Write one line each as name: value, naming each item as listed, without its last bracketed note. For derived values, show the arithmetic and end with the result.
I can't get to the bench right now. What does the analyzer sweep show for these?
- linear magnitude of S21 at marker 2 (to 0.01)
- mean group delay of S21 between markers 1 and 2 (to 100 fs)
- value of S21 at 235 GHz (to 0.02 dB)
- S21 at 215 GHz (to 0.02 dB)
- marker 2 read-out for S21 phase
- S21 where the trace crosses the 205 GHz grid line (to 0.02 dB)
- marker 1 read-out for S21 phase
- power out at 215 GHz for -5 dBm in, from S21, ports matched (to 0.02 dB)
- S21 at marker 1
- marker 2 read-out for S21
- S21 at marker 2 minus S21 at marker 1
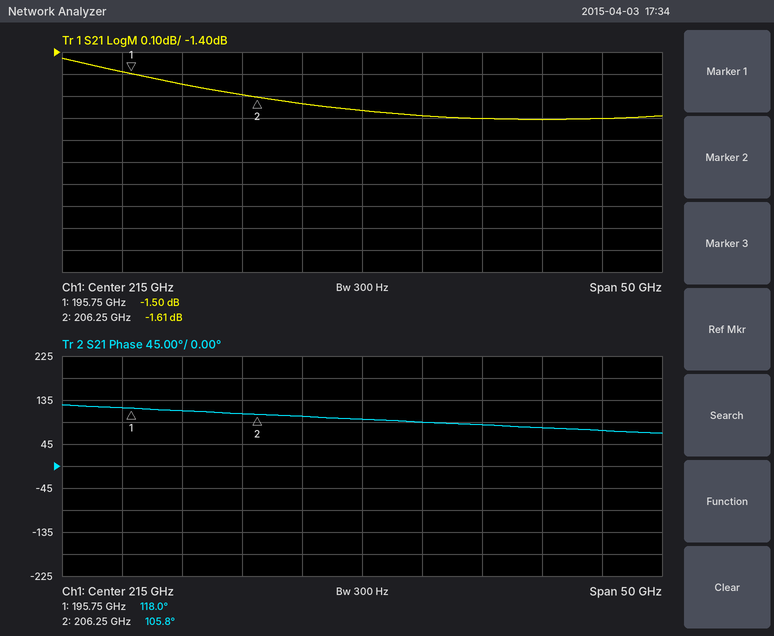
linear magnitude of S21 at marker 2: 10^(-1.61/20) ≈ 0.83
mean group delay of S21 between markers 1 and 2: −(105.8° − (118°))/(360° × 10.5 GHz) ≈ 3.2 ps
value of S21 at 235 GHz: -1.70 dB
S21 at 215 GHz: -1.66 dB
marker 2 read-out for S21 phase: 105.8°
S21 where the trace crosses the 205 GHz grid line: -1.60 dB
marker 1 read-out for S21 phase: 118.0°
power out at 215 GHz for -5 dBm in, from S21, ports matched: -5 dBm + (-1.66 dB) = -6.66 dBm
S21 at marker 1: -1.50 dB
marker 2 read-out for S21: -1.61 dB
S21 at marker 2 minus S21 at marker 1: -1.61 − (-1.5) = -0.11 dB
